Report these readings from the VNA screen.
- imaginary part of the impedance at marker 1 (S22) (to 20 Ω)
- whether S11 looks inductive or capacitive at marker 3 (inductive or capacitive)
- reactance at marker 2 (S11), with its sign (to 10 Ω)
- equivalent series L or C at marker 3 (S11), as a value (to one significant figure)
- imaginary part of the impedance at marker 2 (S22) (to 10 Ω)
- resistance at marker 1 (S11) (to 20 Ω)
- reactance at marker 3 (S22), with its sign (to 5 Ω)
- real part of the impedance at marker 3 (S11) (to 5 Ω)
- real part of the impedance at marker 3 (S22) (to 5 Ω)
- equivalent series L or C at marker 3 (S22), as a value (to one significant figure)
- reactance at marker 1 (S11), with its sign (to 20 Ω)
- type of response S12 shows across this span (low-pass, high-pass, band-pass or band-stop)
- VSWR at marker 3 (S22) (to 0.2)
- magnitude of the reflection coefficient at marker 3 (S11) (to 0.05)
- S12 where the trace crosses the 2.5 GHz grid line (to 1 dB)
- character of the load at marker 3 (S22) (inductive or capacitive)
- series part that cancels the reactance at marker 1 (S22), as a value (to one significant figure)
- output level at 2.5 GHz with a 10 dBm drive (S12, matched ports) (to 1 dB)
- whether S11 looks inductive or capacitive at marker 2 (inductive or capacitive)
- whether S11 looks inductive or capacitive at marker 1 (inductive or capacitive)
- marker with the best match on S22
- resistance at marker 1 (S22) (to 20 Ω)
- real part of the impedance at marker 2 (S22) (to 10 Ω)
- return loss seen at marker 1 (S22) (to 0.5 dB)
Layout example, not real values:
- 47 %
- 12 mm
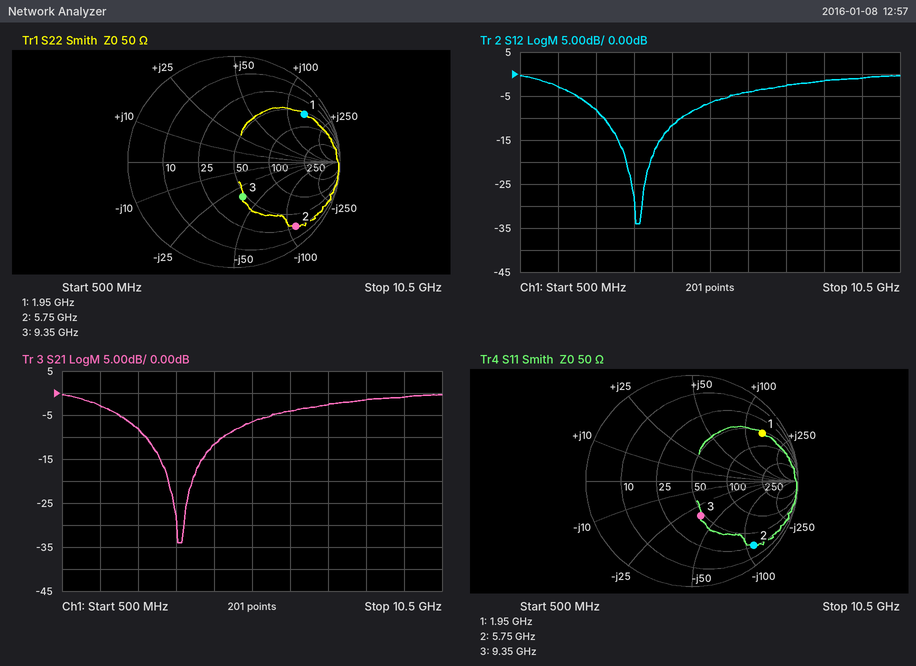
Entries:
- +140 Ω
- capacitive
- -110 Ω
- 500 fF
- -110 Ω
- 60 Ω
- -35 Ω
- 45 Ω
- 45 Ω
- 500 fF
- +140 Ω
- band-stop
- 2.0
- 0.35
- -8 dB
- capacitive
- 600 fF
- 2 dBm
- capacitive
- inductive
- marker 3
- 60 Ω
- 30 Ω
- 2.0 dB
